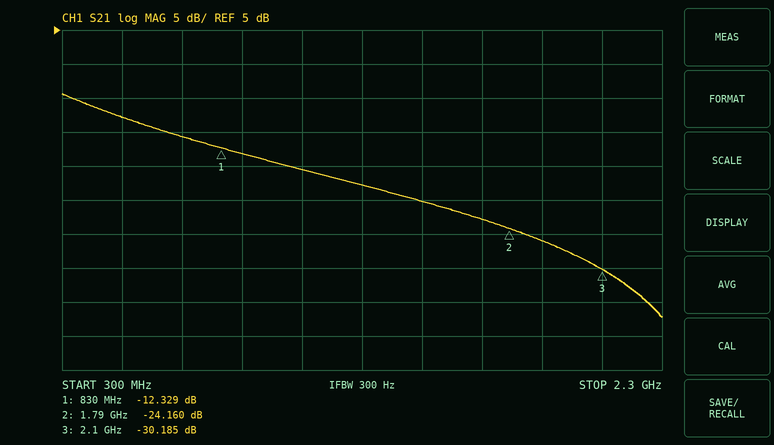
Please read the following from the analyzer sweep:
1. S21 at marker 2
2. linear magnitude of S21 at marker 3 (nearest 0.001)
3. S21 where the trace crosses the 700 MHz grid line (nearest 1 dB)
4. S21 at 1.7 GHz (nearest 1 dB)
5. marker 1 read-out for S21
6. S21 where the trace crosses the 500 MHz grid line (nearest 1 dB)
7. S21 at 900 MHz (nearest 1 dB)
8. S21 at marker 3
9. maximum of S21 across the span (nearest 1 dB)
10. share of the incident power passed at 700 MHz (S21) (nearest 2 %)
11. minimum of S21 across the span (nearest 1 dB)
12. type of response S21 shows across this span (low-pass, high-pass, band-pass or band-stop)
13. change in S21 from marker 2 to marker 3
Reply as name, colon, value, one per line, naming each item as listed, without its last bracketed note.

S21 at marker 2: -24.160 dB
linear magnitude of S21 at marker 3: 0.031
S21 where the trace crosses the 700 MHz grid line: -11 dB
S21 at 1.7 GHz: -23 dB
marker 1 read-out for S21: -12.329 dB
S21 where the trace crosses the 500 MHz grid line: -8 dB
S21 at 900 MHz: -13 dB
S21 at marker 3: -30.185 dB
maximum of S21 across the span: -4 dB
share of the incident power passed at 700 MHz (S21): 8 %
minimum of S21 across the span: -37 dB
type of response S21 shows across this span: low-pass
change in S21 from marker 2 to marker 3: -6.025 dB
